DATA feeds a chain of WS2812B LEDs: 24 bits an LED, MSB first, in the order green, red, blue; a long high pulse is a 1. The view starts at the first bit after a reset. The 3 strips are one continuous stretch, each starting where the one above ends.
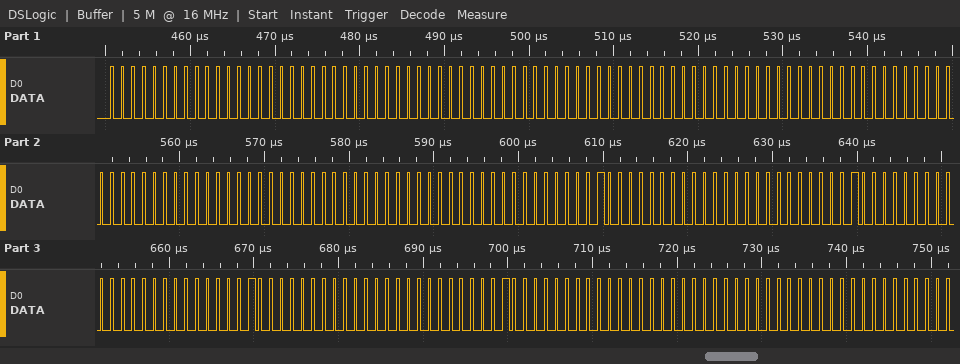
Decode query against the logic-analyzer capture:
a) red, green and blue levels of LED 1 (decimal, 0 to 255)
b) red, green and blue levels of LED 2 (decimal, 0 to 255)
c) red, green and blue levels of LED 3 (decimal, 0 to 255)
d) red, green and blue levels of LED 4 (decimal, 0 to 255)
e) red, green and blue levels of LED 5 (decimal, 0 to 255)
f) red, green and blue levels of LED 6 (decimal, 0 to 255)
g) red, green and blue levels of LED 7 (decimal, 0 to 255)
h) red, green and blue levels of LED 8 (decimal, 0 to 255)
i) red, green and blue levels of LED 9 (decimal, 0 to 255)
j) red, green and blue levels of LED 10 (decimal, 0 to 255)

0, 0, 0
0, 0, 0
0, 0, 0
0, 0, 0
0, 0, 0
0, 1, 0
0, 1, 0
0, 1, 0
0, 1, 0
0, 0, 0
